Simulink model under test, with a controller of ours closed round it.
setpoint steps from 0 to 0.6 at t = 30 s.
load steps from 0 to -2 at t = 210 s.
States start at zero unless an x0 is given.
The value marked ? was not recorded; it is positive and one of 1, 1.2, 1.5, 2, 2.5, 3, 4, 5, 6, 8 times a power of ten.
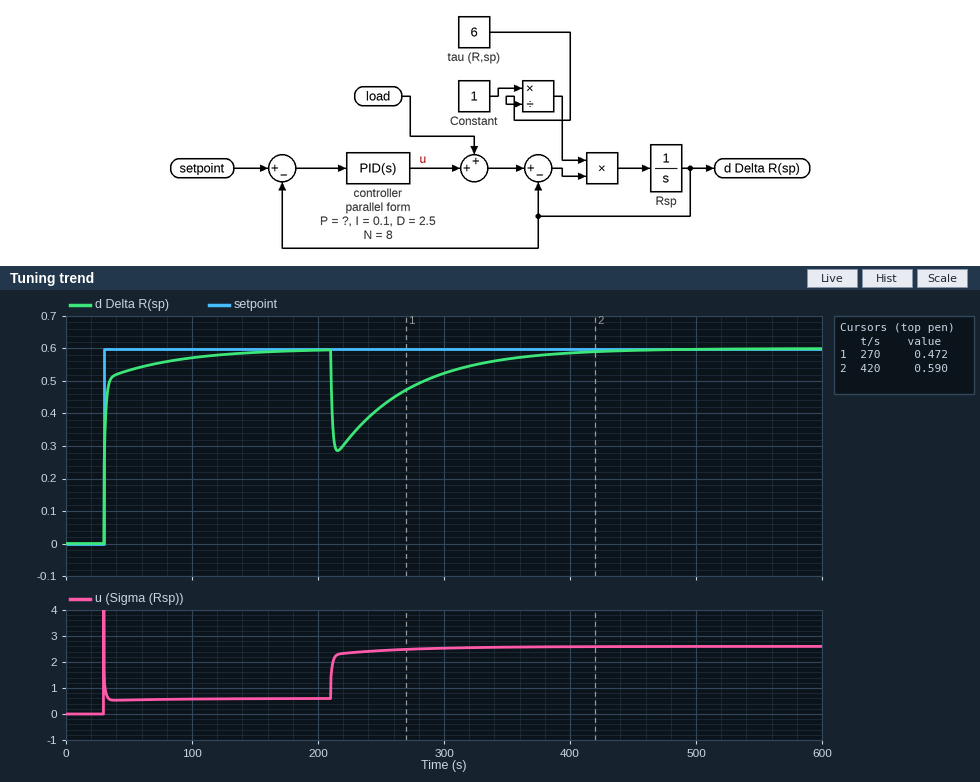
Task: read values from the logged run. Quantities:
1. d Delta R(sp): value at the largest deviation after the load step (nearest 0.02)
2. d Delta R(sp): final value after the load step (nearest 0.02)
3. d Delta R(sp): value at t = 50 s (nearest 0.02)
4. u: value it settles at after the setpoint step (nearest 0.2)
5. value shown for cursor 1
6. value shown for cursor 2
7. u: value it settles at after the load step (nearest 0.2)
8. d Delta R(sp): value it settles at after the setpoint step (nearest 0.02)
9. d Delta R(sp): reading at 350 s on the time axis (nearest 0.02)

0.28
0.60
0.54
0.6
0.472
0.590
2.6
0.60
0.56
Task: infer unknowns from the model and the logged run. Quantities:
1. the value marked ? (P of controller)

5
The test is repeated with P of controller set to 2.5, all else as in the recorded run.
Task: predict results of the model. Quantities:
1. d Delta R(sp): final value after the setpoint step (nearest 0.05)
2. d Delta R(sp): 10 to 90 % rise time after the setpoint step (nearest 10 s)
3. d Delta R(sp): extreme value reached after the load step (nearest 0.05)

0.60
30 s
0.10
